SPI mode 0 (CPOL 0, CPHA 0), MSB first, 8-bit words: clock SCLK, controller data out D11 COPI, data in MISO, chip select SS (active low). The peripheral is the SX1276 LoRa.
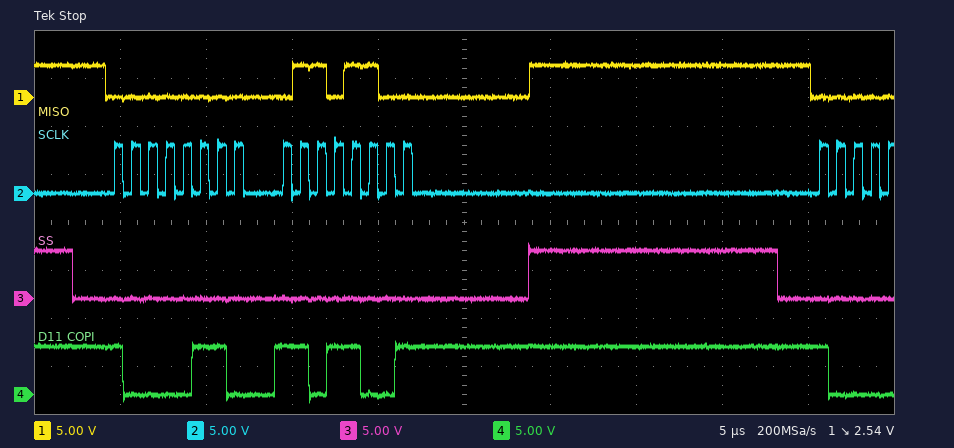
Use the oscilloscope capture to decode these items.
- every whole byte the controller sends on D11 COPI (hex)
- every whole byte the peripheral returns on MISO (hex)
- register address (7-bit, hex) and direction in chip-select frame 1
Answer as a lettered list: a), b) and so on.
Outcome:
a) 0x86 0xD9
b) 0x00 0x6C
c) 0x06 write
